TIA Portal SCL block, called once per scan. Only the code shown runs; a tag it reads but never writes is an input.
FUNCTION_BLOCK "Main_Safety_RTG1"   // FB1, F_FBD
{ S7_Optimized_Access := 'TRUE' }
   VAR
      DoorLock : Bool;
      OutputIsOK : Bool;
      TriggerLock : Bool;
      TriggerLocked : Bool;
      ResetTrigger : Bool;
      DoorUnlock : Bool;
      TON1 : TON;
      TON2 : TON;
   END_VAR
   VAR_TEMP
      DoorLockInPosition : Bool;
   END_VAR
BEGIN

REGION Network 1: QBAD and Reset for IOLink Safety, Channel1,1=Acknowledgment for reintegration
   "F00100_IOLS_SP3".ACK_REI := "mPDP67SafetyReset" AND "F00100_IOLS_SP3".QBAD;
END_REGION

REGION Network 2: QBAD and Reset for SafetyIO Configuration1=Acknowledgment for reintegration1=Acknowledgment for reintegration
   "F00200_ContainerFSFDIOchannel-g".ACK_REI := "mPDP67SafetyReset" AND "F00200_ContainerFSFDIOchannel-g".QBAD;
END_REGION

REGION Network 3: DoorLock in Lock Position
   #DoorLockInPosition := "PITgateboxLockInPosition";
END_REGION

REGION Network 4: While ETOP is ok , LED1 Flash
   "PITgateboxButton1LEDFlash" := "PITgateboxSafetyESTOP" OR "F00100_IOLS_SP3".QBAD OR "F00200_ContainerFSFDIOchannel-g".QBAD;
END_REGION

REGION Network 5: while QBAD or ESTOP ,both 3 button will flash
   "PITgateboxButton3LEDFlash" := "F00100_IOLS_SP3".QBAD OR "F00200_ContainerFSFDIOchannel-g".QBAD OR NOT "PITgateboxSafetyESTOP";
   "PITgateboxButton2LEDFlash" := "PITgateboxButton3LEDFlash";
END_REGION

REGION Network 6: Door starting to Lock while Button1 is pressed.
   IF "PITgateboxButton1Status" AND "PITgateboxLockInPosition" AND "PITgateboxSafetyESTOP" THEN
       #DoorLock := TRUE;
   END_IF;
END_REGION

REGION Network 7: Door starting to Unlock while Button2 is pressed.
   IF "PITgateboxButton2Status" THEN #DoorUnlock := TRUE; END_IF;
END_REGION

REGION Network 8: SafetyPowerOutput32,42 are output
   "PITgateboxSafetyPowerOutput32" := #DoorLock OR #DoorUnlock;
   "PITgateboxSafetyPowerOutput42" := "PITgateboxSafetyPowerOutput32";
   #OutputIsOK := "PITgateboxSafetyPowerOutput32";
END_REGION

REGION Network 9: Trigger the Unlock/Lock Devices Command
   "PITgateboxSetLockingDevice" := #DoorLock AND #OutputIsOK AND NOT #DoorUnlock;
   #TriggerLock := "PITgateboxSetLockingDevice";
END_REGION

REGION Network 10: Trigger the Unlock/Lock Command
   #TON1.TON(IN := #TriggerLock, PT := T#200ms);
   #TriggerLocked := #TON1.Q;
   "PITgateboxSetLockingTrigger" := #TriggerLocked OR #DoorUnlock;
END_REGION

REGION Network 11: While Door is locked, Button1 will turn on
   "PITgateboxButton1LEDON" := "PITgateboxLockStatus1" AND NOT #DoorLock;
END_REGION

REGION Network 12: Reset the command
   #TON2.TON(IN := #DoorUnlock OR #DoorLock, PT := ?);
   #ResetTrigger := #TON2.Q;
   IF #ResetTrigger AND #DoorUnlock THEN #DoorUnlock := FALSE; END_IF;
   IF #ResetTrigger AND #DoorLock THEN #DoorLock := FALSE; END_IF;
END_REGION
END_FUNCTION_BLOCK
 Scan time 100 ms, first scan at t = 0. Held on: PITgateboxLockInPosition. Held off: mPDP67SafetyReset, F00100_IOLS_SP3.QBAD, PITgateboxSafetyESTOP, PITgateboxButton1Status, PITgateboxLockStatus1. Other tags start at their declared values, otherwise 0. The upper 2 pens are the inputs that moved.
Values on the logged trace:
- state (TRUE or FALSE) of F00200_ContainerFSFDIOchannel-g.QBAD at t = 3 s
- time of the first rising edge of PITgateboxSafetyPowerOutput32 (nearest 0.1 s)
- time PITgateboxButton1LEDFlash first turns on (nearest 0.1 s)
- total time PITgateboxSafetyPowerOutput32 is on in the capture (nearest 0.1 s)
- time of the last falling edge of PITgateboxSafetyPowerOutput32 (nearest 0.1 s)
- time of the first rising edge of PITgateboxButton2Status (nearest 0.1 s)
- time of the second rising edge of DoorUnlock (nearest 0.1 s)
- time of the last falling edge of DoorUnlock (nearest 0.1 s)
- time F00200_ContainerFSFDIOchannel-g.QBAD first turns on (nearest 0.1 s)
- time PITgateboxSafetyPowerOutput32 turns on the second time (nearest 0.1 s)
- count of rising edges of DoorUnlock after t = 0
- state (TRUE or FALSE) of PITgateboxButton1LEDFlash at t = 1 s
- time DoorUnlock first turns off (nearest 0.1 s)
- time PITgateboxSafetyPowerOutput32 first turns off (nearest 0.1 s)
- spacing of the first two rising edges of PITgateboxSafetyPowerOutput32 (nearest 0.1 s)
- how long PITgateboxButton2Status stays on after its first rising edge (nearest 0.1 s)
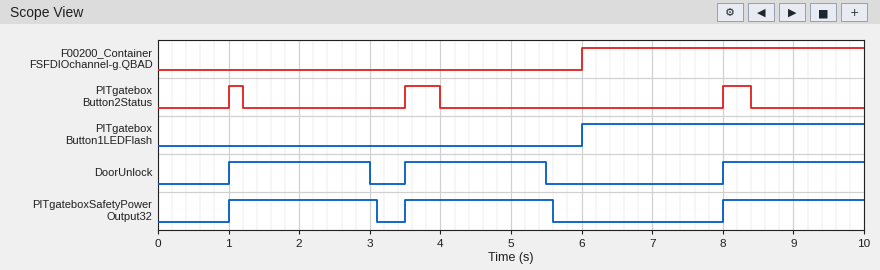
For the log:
FALSE
1.0 s
6.0 s
6.2 s
5.6 s
1.0 s
3.5 s
5.5 s
6.0 s
3.5 s
3
FALSE
3.0 s
3.1 s
2.5 s
0.2 s
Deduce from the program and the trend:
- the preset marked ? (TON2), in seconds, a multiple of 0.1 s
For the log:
2.0 s
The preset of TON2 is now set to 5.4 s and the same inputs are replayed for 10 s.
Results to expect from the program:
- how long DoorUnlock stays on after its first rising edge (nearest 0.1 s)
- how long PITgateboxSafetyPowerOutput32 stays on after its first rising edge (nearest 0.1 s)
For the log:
5.4 s
5.5 s
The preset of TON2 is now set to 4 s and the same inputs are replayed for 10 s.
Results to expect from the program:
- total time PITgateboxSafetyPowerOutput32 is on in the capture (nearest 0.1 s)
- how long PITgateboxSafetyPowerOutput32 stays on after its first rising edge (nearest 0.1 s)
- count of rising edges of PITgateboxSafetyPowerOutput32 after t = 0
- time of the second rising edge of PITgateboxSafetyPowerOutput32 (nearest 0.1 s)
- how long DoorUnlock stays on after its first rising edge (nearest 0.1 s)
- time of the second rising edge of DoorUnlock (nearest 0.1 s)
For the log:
6.1 s
4.1 s
2
8.0 s
4.0 s
8.0 s
